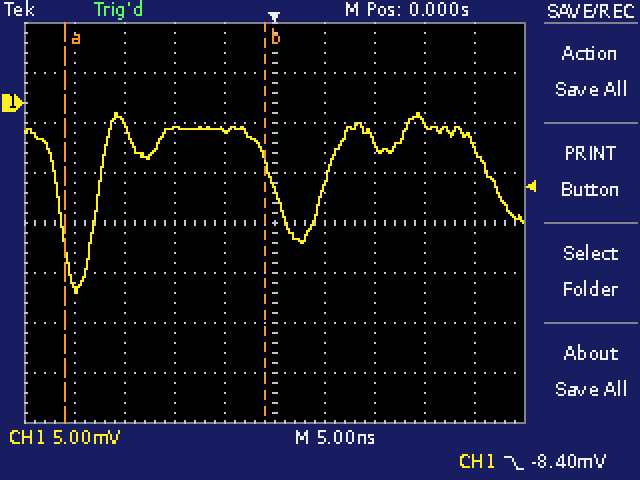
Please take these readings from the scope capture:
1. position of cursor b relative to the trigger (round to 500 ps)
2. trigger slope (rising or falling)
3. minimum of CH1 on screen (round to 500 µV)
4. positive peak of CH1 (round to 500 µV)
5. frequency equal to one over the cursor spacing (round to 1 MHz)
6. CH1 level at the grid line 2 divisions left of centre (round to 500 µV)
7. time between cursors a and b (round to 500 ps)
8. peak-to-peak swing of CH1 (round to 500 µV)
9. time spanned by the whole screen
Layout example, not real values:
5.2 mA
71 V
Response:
-1.0 ns
falling
-19.0 mV
-1.0 mV
50 MHz
-2.5 mV
20.0 ns
18.0 mV
50 ns
